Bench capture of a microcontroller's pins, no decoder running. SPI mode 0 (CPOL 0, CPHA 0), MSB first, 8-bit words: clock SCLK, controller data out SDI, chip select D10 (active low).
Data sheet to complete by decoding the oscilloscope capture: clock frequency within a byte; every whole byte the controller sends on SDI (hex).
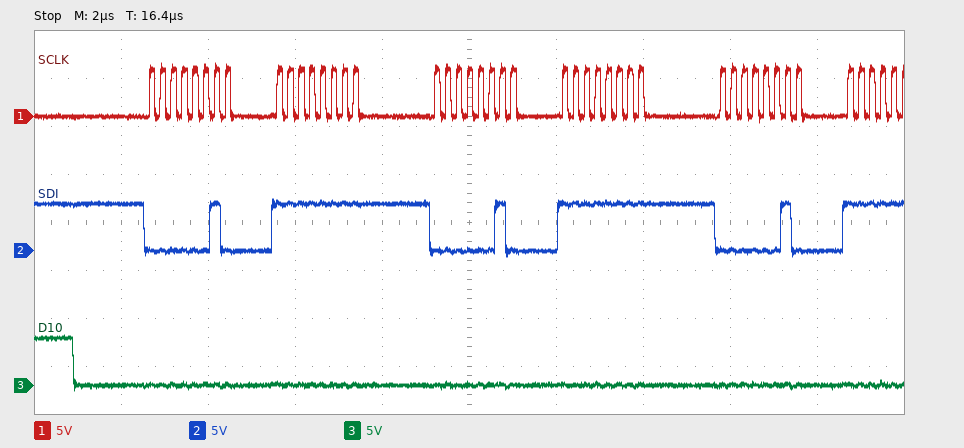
4 MHz
0x02 0xFF 0x02 0xFF 0x02
